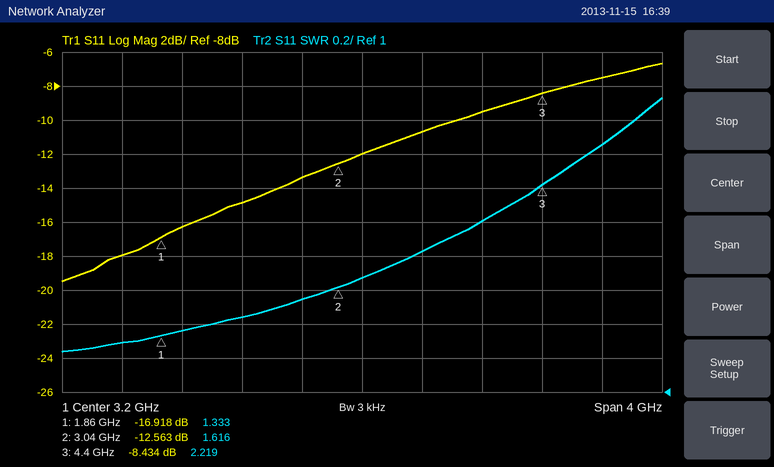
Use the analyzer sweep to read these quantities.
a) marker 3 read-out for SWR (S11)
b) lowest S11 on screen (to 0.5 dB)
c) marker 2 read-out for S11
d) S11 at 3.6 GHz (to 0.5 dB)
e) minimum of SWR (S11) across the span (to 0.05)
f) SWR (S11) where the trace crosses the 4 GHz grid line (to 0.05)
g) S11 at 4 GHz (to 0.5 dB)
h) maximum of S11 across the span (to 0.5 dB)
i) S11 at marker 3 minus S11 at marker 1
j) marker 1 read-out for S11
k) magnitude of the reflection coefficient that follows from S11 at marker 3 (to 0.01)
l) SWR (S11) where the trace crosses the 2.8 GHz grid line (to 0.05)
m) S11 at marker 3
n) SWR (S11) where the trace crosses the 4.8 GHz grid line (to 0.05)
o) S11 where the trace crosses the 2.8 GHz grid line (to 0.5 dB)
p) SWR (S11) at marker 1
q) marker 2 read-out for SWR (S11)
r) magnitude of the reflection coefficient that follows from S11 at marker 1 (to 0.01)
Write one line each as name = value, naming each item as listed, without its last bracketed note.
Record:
marker 3 read-out for SWR = 2.219
lowest S11 on screen = -19.5 dB
marker 2 read-out for S11 = -12.563 dB
S11 at 3.6 GHz = -10.5 dB
minimum of SWR (S11) across the span = 1.25
SWR (S11) where the trace crosses the 4 GHz grid line = 2.00
S11 at 4 GHz = -9.5 dB
maximum of S11 across the span = -6.5 dB
S11 at marker 3 minus S11 at marker 1 = 8.484 dB
marker 1 read-out for S11 = -16.918 dB
magnitude of the reflection coefficient that follows from S11 at marker 3 = 0.38
SWR (S11) where the trace crosses the 2.8 GHz grid line = 1.55
S11 at marker 3 = -8.434 dB
SWR (S11) where the trace crosses the 4.8 GHz grid line = 2.45
S11 where the trace crosses the 2.8 GHz grid line = -13.5 dB
SWR (S11) at marker 1 = 1.333
marker 2 read-out for SWR = 1.616
magnitude of the reflection coefficient that follows from S11 at marker 1 = 0.14
